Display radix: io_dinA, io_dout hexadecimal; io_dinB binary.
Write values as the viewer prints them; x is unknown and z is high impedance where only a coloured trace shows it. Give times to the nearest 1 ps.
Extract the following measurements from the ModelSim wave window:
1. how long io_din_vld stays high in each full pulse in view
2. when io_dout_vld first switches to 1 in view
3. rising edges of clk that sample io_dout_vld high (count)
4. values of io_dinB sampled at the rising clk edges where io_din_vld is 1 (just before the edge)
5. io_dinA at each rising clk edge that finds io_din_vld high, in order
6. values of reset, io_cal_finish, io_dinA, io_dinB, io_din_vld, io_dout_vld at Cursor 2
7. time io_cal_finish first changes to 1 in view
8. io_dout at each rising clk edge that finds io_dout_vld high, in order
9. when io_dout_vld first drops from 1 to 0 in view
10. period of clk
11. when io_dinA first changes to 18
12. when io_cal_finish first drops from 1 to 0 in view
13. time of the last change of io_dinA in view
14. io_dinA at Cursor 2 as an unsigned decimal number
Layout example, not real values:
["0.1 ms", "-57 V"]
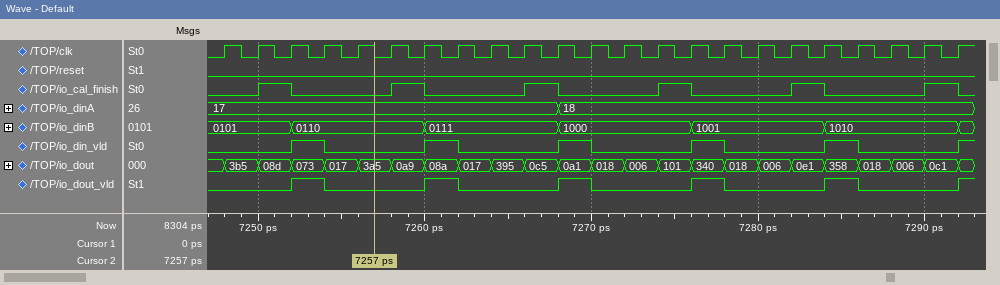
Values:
["2 ps, 2 ps, 2 ps, 2 ps, 2 ps", "7252 ps", "5", "0110, 0111, 1000, 1001, 1010", "17, 17, 18, 18, 18", "reset=0, io_cal_finish=0, io_dinA=17, io_dinB=0110, io_din_vld=0, io_dout_vld=0", "7250 ps", "073, 08a, 0a1, 340, 358", "7254 ps", "2 ps", "7268 ps", "7252 ps", "7268 ps", "23"]
